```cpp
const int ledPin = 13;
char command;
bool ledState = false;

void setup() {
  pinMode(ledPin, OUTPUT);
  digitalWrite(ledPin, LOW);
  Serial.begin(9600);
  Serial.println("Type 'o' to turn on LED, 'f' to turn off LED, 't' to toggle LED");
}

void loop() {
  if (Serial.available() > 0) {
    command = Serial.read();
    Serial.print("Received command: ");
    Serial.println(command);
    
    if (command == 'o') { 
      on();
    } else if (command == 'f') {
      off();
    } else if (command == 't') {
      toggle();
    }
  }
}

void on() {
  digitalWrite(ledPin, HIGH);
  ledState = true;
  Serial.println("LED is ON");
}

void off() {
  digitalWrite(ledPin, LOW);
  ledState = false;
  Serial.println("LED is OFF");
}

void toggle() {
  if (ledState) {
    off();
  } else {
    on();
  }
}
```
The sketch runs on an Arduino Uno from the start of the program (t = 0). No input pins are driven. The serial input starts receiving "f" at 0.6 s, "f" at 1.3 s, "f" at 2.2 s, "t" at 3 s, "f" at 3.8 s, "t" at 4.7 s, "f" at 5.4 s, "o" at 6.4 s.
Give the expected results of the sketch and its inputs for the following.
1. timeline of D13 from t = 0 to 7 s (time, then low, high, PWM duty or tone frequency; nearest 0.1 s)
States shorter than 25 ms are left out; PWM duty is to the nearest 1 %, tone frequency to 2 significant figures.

0 s low; 3 s high; 3.8 s low; 4.7 s high; 5.4 s low; 6.4 s high
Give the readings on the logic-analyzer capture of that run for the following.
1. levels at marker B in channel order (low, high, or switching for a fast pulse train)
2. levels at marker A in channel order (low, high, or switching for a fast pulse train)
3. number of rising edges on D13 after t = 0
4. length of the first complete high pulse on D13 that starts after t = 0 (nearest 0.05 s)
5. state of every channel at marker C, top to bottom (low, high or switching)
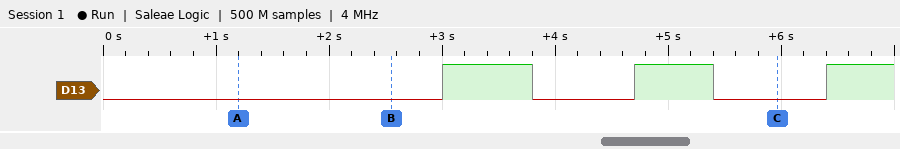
D13 low
D13 low
3
0.80 s
D13 low
